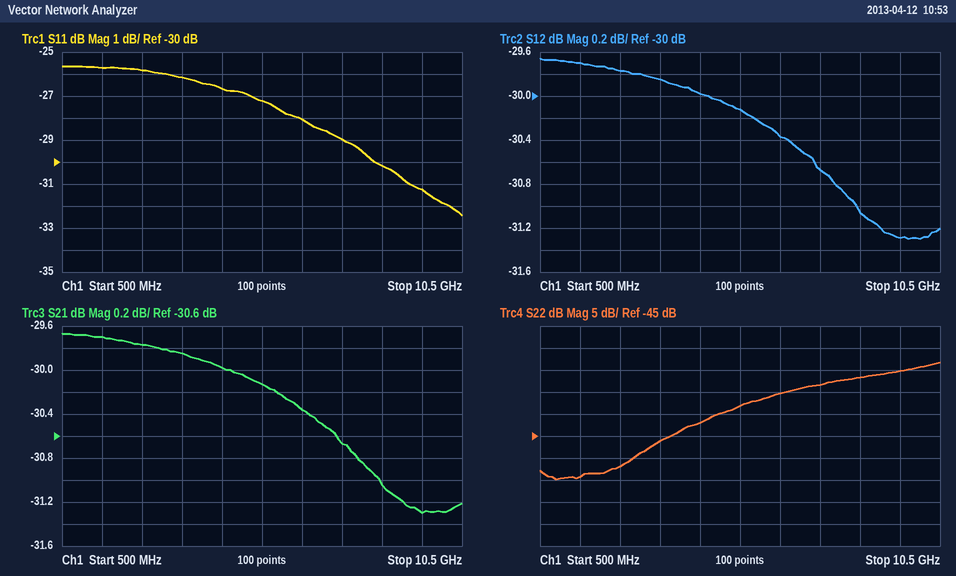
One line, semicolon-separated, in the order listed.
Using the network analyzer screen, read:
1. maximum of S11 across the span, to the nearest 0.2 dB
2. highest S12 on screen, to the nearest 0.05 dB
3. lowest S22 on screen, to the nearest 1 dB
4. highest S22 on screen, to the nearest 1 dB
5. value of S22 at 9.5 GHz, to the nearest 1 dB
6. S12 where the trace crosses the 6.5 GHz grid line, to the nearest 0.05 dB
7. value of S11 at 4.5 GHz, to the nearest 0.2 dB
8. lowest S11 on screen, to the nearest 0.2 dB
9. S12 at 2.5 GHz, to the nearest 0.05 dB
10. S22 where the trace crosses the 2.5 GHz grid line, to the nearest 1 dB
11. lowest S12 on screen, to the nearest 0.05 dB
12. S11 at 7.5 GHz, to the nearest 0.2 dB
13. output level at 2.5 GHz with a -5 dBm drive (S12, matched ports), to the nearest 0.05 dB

-25.6 dB; -29.65 dB; -55 dB; -28 dB; -30 dB; -30.35 dB; -26.6 dB; -32.4 dB; -29.75 dB; -52 dB; -31.30 dB; -29.0 dB; -34.75 dBm
